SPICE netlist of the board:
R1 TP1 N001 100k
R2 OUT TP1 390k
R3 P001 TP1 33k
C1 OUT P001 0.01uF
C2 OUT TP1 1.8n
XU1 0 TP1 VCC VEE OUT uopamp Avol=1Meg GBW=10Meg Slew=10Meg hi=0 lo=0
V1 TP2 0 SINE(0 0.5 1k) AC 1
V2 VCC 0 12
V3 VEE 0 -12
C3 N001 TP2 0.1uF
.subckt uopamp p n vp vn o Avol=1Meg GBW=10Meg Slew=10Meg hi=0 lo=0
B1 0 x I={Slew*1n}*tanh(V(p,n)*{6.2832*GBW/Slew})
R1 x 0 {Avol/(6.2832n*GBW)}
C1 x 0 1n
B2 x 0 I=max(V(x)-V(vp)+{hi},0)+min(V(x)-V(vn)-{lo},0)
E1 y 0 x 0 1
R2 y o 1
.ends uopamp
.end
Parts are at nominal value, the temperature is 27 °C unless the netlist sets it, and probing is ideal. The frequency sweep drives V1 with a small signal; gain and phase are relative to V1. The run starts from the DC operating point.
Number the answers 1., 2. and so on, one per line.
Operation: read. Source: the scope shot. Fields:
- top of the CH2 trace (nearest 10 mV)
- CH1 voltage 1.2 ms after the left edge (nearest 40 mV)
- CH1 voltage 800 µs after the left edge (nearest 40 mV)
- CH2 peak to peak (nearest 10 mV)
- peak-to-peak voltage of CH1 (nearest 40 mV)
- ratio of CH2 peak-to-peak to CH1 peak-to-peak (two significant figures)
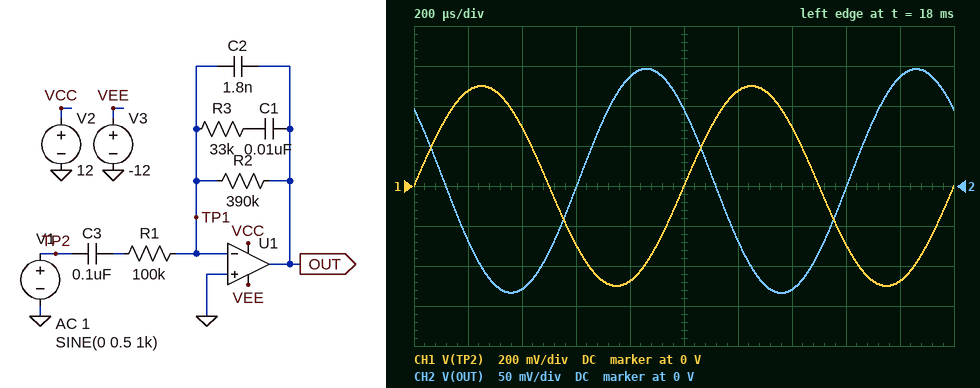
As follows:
1. 150 mV
2. 480 mV
3. -480 mV
4. 280 mV
5. 1.00 V
6. 0.28
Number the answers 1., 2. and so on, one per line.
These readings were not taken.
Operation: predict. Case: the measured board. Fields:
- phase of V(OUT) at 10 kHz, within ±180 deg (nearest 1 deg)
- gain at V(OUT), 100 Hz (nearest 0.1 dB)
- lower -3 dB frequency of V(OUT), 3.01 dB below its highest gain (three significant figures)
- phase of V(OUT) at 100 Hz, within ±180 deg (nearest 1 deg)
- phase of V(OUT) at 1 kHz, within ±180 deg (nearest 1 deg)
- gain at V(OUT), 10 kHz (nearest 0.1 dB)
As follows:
1. 106 deg
2. 1.7 dB
3. 9.03 Hz
4. 127 deg
5. 140 deg
6. -21.5 dB
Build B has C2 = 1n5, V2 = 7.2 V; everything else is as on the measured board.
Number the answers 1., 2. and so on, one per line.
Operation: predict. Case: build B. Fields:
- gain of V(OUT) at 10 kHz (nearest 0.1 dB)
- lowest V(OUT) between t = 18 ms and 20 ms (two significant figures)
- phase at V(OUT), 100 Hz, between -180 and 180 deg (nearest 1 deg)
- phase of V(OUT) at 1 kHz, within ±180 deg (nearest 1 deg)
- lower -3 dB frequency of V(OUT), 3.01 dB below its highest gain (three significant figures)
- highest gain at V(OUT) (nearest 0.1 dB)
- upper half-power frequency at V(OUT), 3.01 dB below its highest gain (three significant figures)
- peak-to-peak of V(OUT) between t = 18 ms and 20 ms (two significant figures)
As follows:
1. -20.1 dB
2. -140 mV
3. 128 deg
4. 143 deg
5. 9.11 Hz
6. 8.4 dB
7. 58.9 Hz
8. 290 mV
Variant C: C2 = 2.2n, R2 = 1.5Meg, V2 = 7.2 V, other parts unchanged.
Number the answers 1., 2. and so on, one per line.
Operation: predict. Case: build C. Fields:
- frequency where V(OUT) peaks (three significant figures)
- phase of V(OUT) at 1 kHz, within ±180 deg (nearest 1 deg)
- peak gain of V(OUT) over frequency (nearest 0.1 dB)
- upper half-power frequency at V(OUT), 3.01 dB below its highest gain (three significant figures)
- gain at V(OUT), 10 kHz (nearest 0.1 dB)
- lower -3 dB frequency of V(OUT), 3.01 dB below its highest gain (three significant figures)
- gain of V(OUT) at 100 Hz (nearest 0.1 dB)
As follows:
1. 11.7 Hz
2. 135 deg
3. 14.4 dB
4. 29.2 Hz
5. -23.1 dB
6. 4.68 Hz
7. 2.2 dB
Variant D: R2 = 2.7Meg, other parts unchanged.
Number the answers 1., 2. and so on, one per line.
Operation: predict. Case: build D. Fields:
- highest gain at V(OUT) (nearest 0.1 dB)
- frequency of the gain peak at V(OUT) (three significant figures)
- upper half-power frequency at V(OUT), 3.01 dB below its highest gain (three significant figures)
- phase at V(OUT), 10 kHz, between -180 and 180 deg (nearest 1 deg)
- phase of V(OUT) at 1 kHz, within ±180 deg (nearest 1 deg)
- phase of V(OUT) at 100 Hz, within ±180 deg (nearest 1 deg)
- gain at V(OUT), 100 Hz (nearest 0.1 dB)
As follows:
1. 16.1 dB
2. 8.88 Hz
3. 24.2 Hz
4. 105 deg
5. 138 deg
6. 112 deg
7. 2.6 dB
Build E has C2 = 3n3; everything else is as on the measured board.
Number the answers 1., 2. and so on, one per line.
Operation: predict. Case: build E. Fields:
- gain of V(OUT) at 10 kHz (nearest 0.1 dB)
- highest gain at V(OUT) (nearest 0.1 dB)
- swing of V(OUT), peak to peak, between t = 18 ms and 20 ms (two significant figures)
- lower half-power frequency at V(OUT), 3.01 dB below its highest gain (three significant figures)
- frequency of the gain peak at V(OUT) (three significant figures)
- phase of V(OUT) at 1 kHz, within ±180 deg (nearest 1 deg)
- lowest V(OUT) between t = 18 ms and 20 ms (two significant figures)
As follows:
1. -26.5 dB
2. 8.1 dB
3. 240 mV
4. 8.66 Hz
5. 21.6 Hz
6. 131 deg
7. -110 mV
